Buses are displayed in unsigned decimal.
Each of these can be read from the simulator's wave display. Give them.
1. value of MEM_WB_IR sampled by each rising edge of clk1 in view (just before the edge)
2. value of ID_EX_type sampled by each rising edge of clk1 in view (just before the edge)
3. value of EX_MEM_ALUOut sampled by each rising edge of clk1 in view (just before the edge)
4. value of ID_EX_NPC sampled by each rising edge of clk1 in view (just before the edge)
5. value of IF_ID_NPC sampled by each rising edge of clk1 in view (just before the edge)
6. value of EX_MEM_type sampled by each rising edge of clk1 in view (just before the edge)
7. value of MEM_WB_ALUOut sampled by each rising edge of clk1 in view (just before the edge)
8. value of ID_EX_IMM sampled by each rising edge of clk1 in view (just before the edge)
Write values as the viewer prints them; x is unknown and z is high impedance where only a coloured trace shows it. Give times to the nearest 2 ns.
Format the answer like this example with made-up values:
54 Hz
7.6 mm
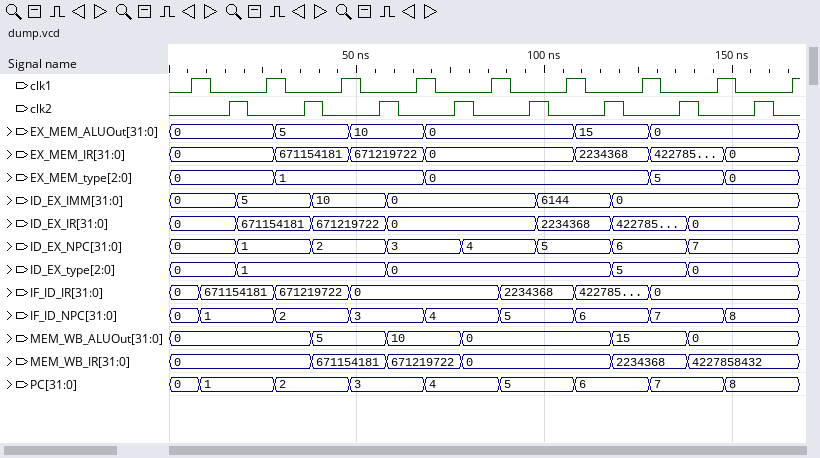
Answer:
0, 0, 671154181, 671219722, 0, 0, 2234368, 4227858432, 4227858432
0, 1, 1, 0, 0, 0, 5, 0, 0
0, 0, 5, 10, 0, 0, 15, 0, 0
0, 1, 2, 3, 4, 5, 6, 7, 7
0, 1, 2, 3, 4, 5, 6, 7, 8
0, 0, 1, 1, 0, 0, 0, 5, 0
0, 0, 5, 10, 0, 0, 15, 0, 0
0, 5, 10, 0, 0, 6144, 0, 0, 0
